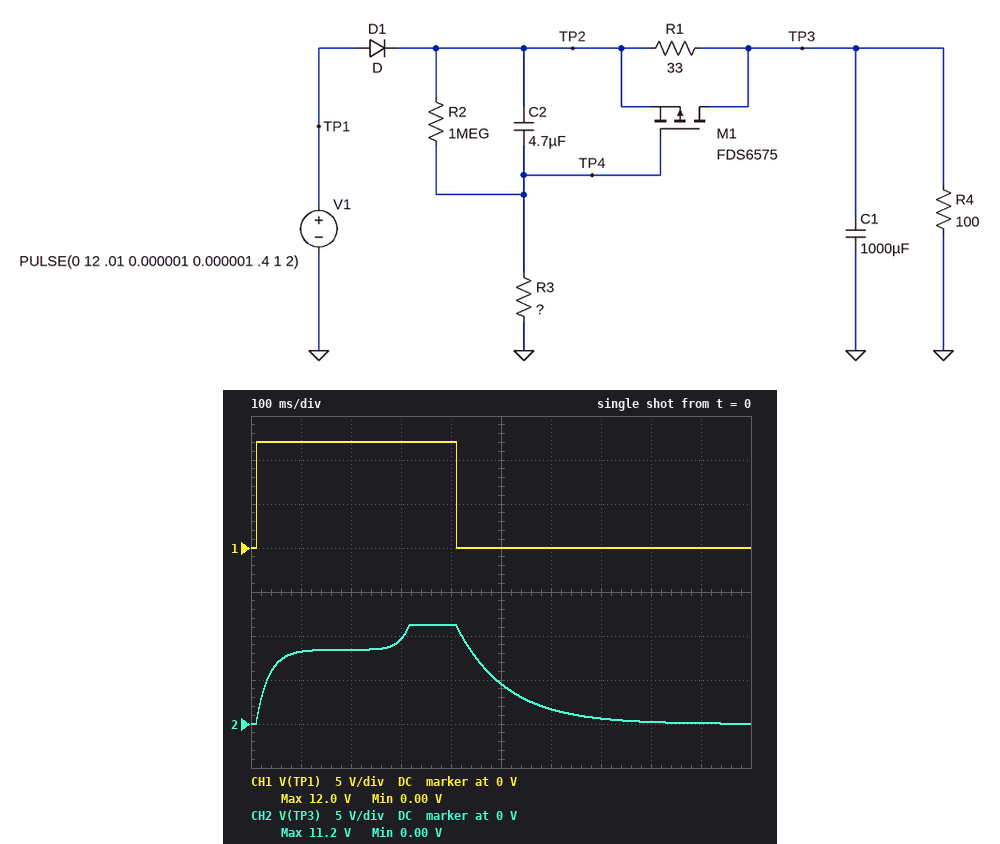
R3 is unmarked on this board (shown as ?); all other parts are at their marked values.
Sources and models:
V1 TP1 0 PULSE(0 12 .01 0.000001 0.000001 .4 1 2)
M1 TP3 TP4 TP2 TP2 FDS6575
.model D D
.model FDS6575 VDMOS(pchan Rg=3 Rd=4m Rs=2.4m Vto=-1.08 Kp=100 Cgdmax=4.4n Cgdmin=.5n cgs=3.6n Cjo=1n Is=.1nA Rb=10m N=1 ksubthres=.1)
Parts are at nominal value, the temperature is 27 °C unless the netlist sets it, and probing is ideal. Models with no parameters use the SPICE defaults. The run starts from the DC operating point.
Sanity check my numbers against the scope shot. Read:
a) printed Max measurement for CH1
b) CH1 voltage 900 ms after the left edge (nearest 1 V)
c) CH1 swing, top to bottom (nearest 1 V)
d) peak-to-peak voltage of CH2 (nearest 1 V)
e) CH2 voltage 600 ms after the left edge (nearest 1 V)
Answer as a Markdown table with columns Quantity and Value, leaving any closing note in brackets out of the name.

| Quantity | Value |
|---|---|
| printed Max measurement for CH1 | 12.0 V |
| CH1 voltage 900 ms after the left edge | 0 V |
| CH1 swing, top to bottom | 12 V |
| peak-to-peak voltage of CH2 | 11 V |
| CH2 voltage 600 ms after the left edge | 2 V |
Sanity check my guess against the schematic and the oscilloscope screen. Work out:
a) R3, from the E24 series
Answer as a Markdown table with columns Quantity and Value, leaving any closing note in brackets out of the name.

| Quantity | Value |
|---|---|
| R3, from the E24 series | 620 kΩ |
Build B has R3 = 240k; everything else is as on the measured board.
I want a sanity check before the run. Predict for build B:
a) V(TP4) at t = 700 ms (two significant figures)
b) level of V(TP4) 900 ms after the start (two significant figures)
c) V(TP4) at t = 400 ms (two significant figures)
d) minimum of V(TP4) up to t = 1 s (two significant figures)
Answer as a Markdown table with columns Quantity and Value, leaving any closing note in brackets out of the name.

| Quantity | Value |
|---|---|
| V(TP4) at t = 700 ms | -2.5 V |
| level of V(TP4) 900 ms after the start | -2.4 V |
| V(TP4) at t = 400 ms | 8.1 V |
| minimum of V(TP4) up to t = 1 s | -2.6 V |
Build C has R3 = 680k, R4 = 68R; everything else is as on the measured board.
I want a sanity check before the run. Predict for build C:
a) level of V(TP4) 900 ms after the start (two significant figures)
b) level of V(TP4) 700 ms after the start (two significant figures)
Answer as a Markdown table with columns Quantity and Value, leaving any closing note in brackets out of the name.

| Quantity | Value |
|---|---|
| level of V(TP4) 900 ms after the start | -1.2 V |
| level of V(TP4) 700 ms after the start | -1.1 V |
